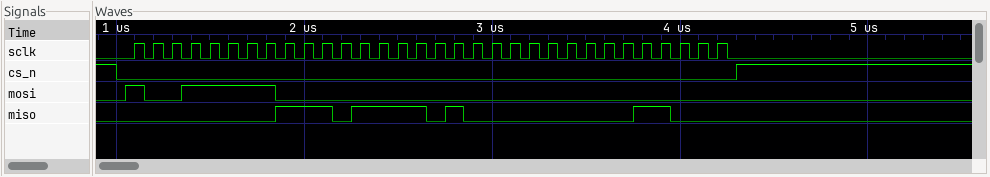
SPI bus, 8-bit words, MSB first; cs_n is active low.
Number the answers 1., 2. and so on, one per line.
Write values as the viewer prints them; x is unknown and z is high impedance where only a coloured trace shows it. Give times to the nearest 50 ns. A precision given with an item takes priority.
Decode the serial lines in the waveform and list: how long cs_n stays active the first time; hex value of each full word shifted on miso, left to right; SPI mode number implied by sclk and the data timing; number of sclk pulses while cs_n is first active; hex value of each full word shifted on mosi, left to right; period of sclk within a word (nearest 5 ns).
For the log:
1. 3300 ns
2. 00, EF, 40, 18
3. 0
4. 32
5. 9F, 00, 00, 00
6. 100 ns
